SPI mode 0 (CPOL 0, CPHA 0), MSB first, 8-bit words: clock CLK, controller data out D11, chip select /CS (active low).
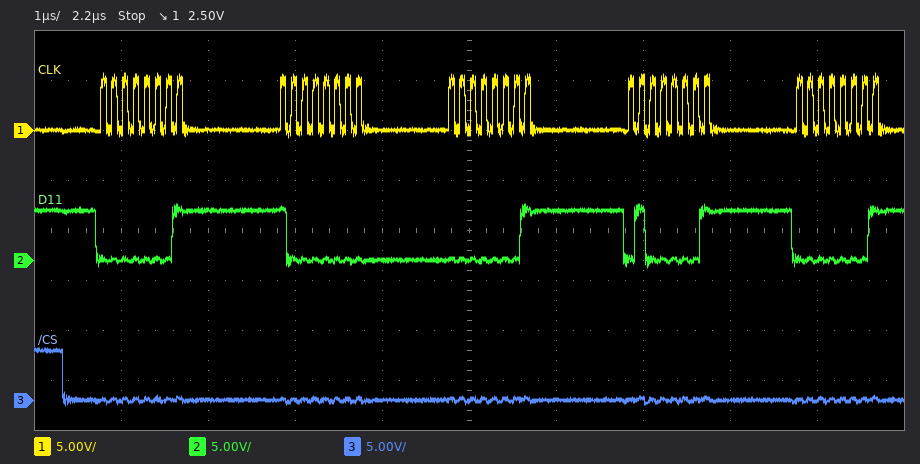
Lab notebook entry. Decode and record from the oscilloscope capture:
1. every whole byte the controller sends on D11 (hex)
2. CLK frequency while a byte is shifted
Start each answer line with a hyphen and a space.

- 01 80 01 41 01
- 8 MHz
